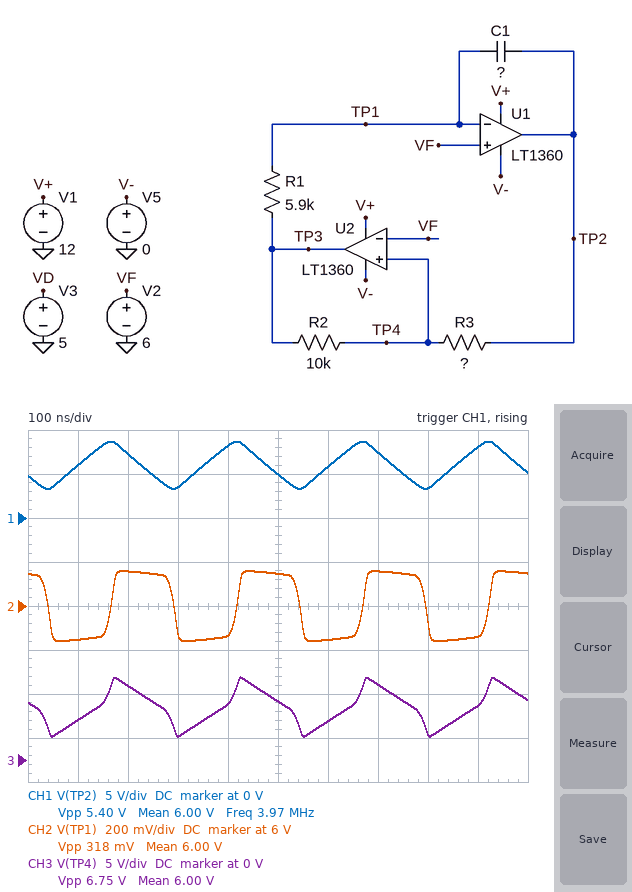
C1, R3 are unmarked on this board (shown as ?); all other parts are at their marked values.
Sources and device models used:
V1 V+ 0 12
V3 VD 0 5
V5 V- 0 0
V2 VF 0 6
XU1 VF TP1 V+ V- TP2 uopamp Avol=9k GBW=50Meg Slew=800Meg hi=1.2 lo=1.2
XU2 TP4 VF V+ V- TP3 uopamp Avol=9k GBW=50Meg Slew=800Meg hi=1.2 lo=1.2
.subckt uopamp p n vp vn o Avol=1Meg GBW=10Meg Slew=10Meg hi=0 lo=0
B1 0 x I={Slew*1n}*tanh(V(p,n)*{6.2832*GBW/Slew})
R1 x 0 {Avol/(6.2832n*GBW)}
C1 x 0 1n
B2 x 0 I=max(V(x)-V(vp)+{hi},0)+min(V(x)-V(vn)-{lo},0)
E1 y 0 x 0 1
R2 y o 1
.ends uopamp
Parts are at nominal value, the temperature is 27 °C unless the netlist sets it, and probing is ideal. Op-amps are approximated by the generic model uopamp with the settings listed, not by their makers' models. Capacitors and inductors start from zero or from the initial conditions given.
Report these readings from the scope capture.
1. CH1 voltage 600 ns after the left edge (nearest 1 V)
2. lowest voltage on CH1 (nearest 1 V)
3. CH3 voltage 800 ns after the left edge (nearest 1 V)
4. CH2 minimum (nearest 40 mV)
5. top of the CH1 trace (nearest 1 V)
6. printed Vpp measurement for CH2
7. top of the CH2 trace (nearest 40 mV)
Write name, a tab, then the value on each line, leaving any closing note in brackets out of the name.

CH1 voltage 600 ns after the left edge	6 V
lowest voltage on CH1	3 V
CH3 voltage 800 ns after the left edge	3 V
CH2 minimum	5.84 V
top of the CH1 trace	9 V
printed Vpp measurement for CH2	318 mV
top of the CH2 trace	6.16 V
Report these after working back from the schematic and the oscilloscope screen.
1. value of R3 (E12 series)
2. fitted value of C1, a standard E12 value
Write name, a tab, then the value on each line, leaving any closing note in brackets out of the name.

value of R3	3.9 kΩ
fitted value of C1, a standard E12 value	18 pF
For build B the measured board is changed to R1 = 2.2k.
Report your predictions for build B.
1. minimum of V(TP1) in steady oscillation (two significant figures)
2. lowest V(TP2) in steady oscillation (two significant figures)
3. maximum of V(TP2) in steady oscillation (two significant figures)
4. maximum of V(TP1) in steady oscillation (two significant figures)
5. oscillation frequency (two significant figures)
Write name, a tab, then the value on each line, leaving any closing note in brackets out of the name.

minimum of V(TP1) in steady oscillation	5.6 V
lowest V(TP2) in steady oscillation	2.6 V
maximum of V(TP2) in steady oscillation	9.4 V
maximum of V(TP1) in steady oscillation	6.4 V
oscillation frequency	7.5 MHz
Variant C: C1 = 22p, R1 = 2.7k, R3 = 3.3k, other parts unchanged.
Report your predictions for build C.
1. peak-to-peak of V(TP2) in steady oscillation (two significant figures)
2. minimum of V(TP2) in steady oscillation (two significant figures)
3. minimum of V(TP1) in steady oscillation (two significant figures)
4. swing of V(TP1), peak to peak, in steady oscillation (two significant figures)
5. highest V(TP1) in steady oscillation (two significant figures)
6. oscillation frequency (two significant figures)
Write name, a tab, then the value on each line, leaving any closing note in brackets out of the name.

peak-to-peak of V(TP2) in steady oscillation	5.6 V
minimum of V(TP2) in steady oscillation	3.2 V
minimum of V(TP1) in steady oscillation	5.7 V
swing of V(TP1), peak to peak, in steady oscillation	550 mV
highest V(TP1) in steady oscillation	6.3 V
oscillation frequency	6.3 MHz
